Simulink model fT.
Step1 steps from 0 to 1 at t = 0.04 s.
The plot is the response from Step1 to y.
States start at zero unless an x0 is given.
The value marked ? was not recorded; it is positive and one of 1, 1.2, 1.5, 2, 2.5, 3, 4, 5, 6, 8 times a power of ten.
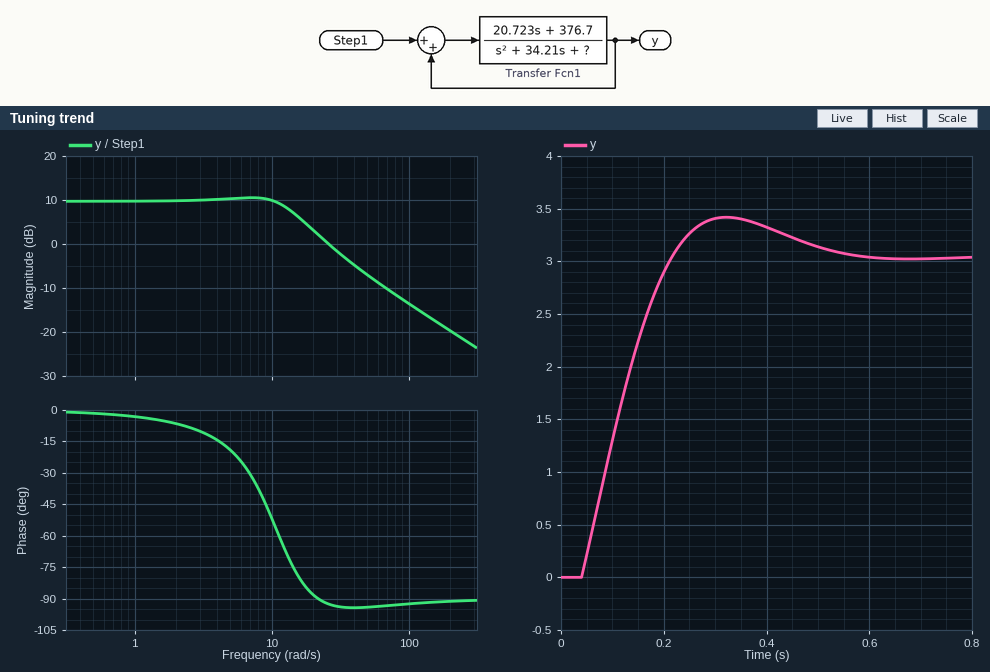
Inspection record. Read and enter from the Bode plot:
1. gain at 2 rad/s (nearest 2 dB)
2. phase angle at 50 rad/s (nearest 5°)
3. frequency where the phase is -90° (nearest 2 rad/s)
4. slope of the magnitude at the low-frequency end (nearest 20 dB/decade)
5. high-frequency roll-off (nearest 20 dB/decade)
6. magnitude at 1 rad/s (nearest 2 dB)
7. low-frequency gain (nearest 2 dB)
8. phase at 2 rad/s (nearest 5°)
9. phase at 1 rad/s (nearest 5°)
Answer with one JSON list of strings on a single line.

["10 dB", "-95°", "22 rad/s", "0 dB/decade", "-20 dB/decade", "10 dB", "10 dB", "-5°", "-5°"]
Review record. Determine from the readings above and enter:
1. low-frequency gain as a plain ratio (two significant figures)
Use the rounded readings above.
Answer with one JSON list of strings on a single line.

["3.2"]
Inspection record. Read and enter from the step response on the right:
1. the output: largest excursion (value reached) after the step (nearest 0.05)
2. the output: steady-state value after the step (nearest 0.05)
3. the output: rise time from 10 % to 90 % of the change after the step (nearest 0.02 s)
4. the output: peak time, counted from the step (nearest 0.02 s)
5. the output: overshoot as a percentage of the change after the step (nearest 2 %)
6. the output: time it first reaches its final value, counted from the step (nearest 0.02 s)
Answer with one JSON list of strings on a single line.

["3.40", "3.05", "0.14 s", "0.28 s", "12 %", "0.18 s"]
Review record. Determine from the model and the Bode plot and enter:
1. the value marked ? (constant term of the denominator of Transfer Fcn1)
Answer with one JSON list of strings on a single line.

["500"]
